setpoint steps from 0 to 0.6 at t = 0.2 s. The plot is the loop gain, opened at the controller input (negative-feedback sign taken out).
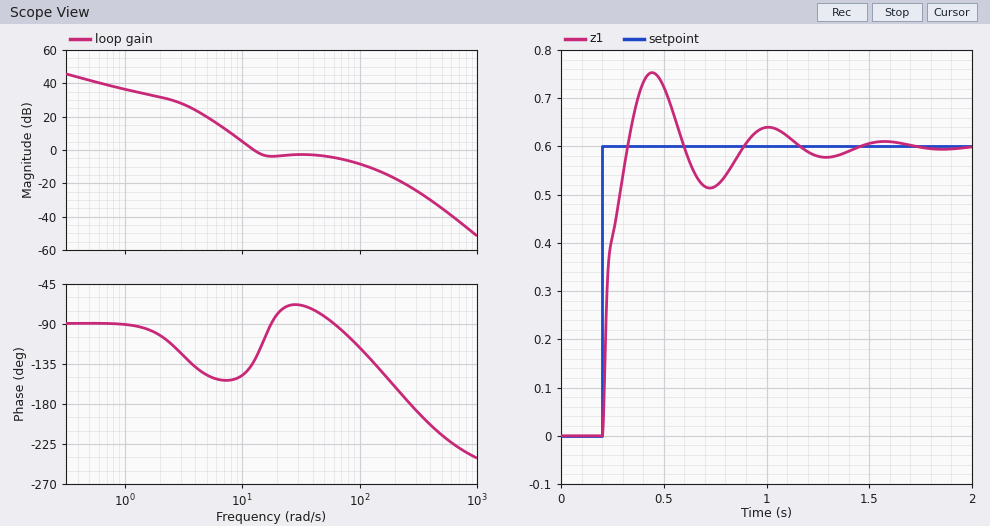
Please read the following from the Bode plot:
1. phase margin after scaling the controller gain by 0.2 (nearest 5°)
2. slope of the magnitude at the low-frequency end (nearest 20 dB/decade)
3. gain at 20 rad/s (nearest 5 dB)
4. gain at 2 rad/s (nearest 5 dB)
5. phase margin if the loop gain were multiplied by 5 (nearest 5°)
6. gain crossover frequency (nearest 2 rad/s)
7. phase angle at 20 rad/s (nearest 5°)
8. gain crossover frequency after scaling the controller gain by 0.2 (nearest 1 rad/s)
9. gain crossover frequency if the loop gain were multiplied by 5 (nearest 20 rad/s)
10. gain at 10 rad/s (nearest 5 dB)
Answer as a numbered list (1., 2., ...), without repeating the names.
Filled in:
1. 25°
2. -20 dB/decade
3. -5 dB
4. 30 dB
5. 35°
6. 12 rad/s
7. -80°
8. 7 rad/s
9. 160 rad/s
10. 5 dB
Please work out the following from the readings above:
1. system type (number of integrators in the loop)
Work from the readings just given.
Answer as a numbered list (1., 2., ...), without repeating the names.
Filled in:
1. 1
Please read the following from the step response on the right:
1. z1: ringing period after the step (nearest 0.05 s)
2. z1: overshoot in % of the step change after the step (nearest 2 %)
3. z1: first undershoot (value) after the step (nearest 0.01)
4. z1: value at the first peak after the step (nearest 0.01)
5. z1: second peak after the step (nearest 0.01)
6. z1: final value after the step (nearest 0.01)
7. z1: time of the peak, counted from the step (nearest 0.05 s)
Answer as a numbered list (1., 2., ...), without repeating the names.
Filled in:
1. 0.55 s
2. 26 %
3. 0.51
4. 0.75
5. 0.64
6. 0.60
7. 0.25 s
